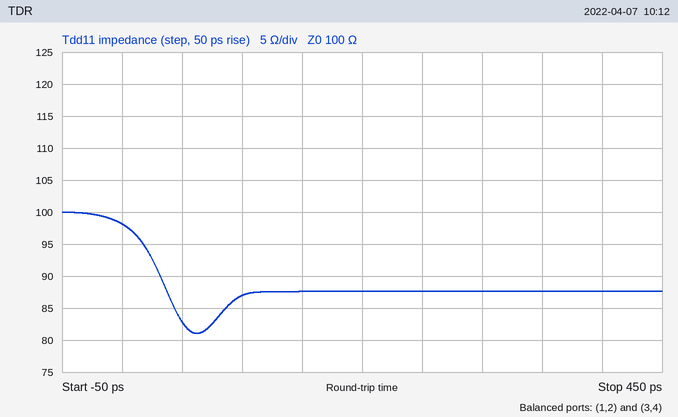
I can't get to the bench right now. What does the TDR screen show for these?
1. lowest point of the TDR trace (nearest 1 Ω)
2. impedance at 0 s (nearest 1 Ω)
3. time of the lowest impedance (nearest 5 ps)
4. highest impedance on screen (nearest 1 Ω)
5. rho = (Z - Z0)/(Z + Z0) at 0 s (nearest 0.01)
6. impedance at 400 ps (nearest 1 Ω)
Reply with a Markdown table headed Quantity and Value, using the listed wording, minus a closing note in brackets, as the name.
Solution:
| Quantity | Value |
|---|---|
| lowest point of the TDR trace | 81 Ω |
| impedance at 0 s | 98 Ω |
| time of the lowest impedance | 60 ps |
| highest impedance on screen | 100 Ω |
| rho = (Z - Z0)/(Z + Z0) at 0 s | -0.01 |
| impedance at 400 ps | 88 Ω |
